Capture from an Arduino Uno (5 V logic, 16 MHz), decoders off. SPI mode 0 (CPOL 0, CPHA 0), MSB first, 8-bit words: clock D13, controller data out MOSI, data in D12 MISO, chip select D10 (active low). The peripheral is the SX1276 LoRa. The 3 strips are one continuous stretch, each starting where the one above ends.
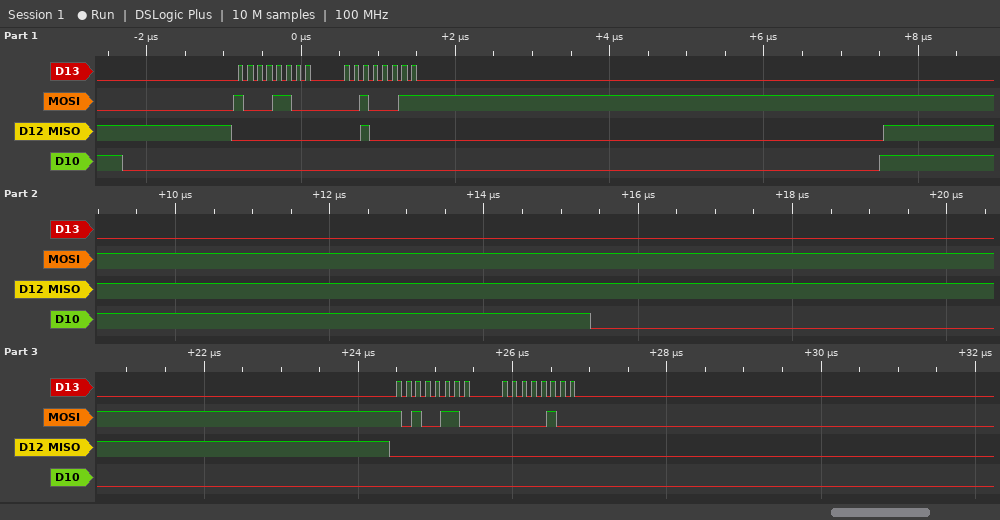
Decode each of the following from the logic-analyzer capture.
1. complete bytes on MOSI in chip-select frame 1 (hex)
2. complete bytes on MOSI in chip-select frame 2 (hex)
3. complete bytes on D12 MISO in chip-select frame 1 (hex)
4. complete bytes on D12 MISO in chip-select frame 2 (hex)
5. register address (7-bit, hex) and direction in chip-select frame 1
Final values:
8C 23
A6 04
00 20
00 00
0x0C write
